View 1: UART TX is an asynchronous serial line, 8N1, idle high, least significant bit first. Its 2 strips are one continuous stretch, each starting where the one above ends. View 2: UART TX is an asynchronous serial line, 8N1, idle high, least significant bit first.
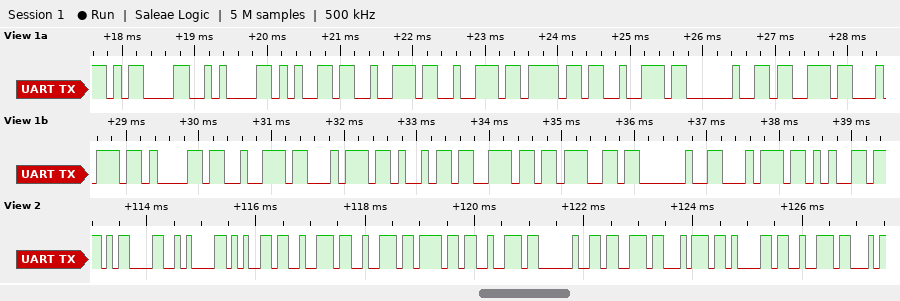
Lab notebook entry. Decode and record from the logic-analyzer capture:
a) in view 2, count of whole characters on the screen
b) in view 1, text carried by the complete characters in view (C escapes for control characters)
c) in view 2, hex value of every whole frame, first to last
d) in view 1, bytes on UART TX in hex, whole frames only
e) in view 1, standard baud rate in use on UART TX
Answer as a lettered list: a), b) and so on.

a) 12
b) "\r\nerror starting te"
c) 0x0D 0x0A 0x65 0x72 0x72 0x6F 0x72 0x20 0x73 0x74 0x61 0x72
d) 0D 0A 65 72 72 6F 72 20 73 74 61 72 74 69 6E 67 20 74 65
e) 9600 baud
